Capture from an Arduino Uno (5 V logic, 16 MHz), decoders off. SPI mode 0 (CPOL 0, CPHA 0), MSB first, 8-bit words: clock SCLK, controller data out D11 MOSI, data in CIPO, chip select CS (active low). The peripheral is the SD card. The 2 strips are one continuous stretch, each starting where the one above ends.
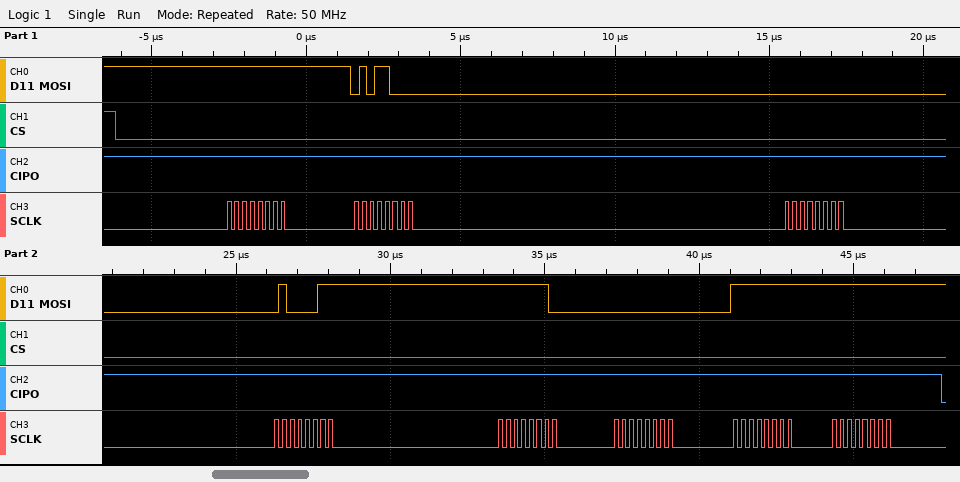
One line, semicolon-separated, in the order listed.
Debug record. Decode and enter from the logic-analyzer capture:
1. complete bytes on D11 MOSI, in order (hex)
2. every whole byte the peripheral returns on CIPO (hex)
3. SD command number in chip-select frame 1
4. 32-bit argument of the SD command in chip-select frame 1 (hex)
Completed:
FF 58 00 43 FE 00 FF FF; FF FF FF FF FF FF FF FF; CMD24; 0x0043FE00
